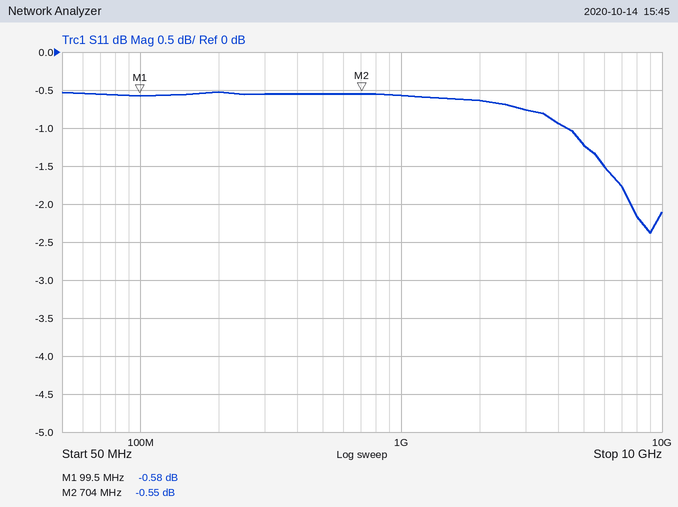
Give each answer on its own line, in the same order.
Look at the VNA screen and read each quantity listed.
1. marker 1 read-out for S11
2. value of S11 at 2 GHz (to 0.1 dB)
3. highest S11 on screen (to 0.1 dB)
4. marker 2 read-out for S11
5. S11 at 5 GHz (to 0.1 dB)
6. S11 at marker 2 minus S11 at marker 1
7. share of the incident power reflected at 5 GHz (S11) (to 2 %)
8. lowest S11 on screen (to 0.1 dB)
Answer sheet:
-0.58 dB
-0.6 dB
-0.5 dB
-0.55 dB
-1.2 dB
0.03 dB
76 %
-2.4 dB
